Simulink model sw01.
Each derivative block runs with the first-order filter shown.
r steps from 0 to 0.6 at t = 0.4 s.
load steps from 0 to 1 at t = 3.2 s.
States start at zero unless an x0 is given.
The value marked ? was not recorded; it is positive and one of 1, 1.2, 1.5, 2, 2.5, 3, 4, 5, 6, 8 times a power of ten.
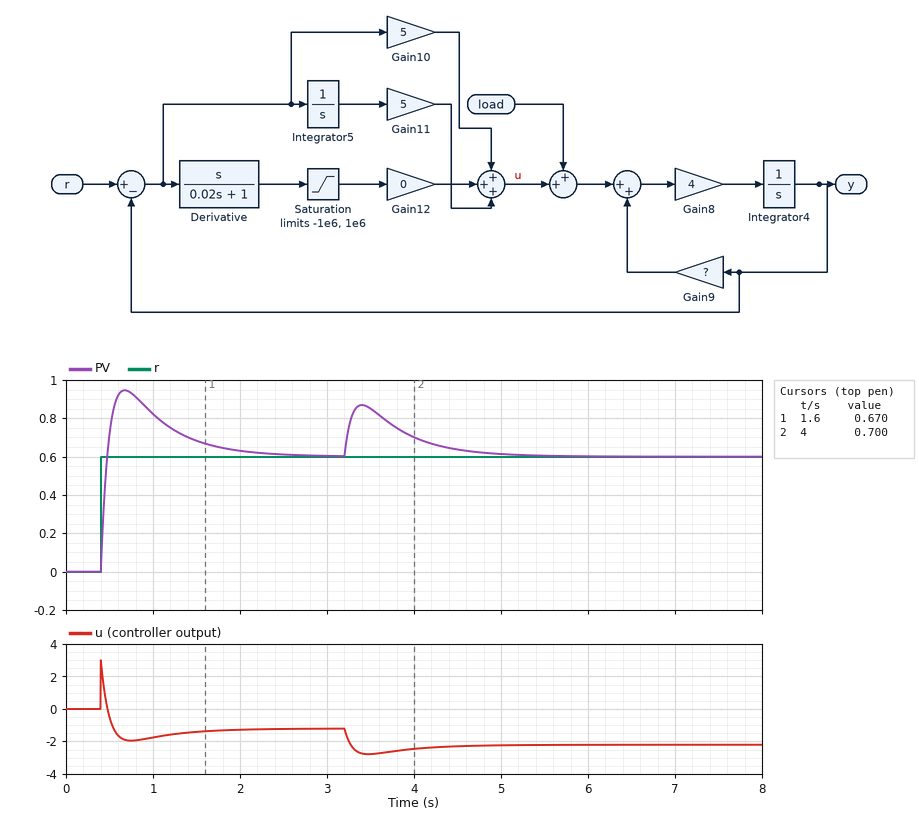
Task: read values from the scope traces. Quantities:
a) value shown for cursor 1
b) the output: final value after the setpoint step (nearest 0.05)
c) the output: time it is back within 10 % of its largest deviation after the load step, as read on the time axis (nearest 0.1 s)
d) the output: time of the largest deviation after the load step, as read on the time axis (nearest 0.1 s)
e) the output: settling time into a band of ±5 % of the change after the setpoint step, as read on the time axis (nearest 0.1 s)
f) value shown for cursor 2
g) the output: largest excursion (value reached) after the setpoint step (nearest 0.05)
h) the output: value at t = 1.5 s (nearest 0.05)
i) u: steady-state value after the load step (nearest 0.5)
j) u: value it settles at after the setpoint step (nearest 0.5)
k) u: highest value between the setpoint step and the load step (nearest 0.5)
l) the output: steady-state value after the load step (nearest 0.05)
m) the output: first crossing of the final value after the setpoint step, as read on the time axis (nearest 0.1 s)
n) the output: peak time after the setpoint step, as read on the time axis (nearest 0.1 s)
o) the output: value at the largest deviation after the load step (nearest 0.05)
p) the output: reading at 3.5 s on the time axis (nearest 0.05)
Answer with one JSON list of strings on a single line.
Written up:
["0.670", "0.60", "4.7 s", "3.4 s", "2.0 s", "0.700", "0.95", "0.70", "-2.0", "-1.0", "3.0", "0.60", "0.5 s", "0.7 s", "0.85", "0.85"]
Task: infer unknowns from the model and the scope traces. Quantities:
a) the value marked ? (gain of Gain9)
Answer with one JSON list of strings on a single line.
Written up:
["2"]
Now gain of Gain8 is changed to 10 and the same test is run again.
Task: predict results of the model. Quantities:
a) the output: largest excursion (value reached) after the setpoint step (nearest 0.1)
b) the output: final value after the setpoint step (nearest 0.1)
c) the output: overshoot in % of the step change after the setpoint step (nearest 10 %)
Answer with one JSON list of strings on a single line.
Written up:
["1.0", "0.6", "60 %"]
